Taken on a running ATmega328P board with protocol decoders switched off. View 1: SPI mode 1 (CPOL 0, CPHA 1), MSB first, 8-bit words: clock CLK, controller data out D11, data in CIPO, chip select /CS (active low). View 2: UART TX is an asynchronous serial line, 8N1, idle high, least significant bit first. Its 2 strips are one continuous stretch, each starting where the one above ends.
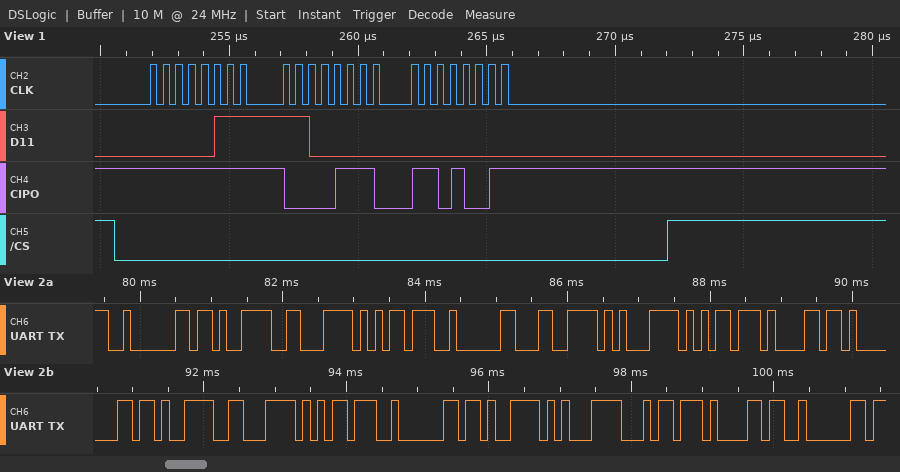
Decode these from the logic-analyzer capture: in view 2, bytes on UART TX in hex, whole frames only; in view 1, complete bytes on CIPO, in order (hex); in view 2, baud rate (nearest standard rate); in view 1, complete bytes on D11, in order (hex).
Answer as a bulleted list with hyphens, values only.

- 0x02 0xCB 0xC6 0xB5 0x02 0xCC 0xC5 0xB5 0x61 0x01 0xCB 0xC6 0xB5 0x02 0xCB 0xC5 0xB4 0x61 0x02
- FF 0E D3
- 9600 baud
- 07 C0 00
